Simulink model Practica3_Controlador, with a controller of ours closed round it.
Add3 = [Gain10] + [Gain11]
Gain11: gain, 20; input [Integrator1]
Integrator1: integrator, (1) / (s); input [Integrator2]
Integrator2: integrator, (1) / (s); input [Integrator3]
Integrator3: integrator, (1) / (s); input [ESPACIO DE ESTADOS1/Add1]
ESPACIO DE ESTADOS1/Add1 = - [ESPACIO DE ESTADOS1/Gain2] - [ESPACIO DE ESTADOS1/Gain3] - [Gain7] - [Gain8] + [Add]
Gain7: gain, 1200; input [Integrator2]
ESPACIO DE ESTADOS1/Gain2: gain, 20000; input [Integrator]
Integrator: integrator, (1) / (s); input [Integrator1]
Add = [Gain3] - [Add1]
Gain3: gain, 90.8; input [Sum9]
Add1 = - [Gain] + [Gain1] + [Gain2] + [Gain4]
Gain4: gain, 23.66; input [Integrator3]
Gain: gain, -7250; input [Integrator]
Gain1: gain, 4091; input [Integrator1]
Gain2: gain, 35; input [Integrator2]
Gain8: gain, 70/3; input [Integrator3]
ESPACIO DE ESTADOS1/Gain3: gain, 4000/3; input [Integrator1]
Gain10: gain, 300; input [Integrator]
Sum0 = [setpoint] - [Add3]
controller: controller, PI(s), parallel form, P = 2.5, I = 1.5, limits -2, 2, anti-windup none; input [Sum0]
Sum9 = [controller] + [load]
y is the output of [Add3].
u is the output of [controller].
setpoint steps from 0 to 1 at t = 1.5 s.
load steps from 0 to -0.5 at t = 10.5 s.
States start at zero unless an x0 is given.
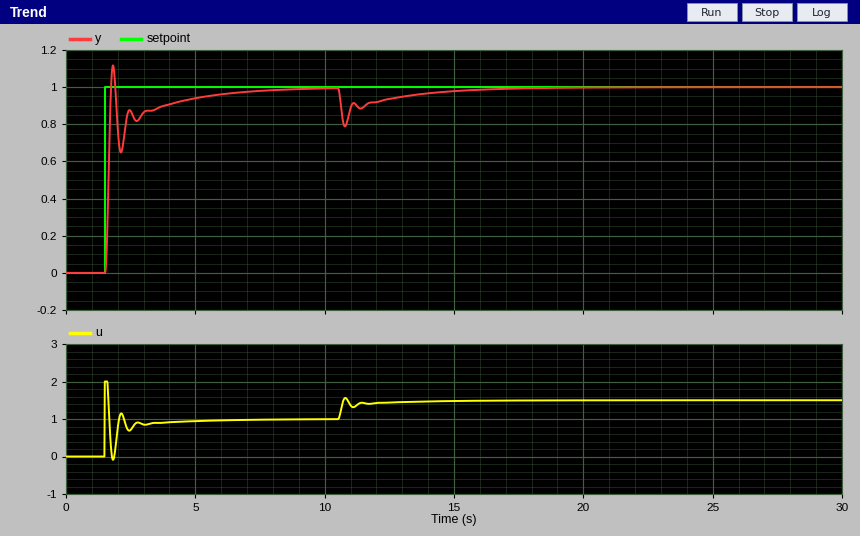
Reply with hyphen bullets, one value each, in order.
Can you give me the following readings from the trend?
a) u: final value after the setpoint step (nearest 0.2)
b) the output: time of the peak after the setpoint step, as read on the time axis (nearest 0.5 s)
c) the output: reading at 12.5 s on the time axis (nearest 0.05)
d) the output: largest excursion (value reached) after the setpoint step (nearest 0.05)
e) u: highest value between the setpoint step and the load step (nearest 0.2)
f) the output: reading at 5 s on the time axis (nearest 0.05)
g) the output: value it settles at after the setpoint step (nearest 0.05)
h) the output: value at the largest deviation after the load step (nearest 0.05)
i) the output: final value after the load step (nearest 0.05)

- 1.0
- 2.0 s
- 0.95
- 1.10
- 2.0
- 0.95
- 1.00
- 0.80
- 1.00
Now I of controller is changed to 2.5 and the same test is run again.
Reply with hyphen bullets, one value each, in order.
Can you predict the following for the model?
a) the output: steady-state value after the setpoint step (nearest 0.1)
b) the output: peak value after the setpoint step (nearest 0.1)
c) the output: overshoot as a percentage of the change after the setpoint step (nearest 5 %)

- 1.0
- 1.2
- 15 %
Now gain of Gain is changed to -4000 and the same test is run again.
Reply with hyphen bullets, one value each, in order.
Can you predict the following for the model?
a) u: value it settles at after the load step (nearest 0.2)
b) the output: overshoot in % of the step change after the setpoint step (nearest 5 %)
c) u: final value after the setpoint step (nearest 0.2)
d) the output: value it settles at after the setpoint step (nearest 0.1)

- 1.4
- 15 %
- 0.8
- 1.0
